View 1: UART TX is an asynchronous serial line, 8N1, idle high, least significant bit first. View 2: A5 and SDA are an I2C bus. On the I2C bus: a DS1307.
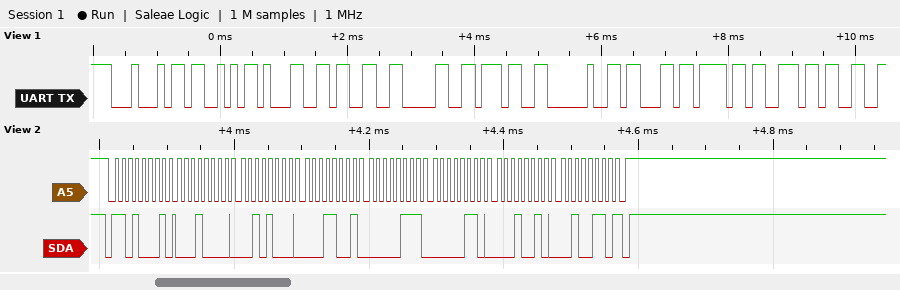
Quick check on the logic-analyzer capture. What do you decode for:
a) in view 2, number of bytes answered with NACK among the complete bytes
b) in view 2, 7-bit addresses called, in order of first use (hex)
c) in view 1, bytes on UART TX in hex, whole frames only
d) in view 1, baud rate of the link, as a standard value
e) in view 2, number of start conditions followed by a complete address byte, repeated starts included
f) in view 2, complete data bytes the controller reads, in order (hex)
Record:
1
0x68
44 53 31 33 30 37 20 63 6F 6E
9600 baud
1
10 28 19 07 06 12 26
